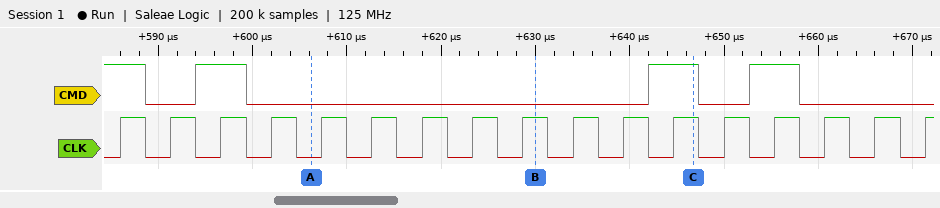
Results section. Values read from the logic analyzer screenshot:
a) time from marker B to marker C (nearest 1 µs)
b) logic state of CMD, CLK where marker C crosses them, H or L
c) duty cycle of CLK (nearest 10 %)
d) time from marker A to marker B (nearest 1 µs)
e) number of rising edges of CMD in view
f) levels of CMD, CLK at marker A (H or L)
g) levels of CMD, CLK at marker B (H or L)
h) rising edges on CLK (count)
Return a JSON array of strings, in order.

["17 µs", "CMD=H, CLK=H", "50 %", "24 µs", "3", "CMD=L, CLK=L", "CMD=L, CLK=H", "17"]
